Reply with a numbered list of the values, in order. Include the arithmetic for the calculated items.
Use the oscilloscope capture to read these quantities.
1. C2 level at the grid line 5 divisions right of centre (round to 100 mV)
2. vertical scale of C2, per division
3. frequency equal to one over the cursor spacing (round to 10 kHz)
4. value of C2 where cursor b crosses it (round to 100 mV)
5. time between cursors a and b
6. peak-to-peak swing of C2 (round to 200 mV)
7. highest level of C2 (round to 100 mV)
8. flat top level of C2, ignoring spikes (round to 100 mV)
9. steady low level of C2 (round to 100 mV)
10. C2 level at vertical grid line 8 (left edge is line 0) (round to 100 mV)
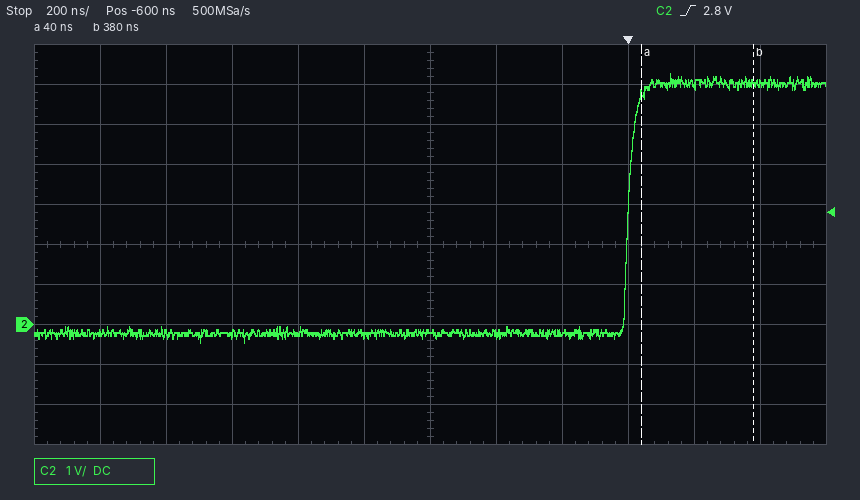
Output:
1. 6.0 V
2. 1 V
3. 1 / 340 ns ≈ 2.94 MHz
4. 6.0 V
5. 380 ns − (40 ns) = 340 ns
6. 6.8 V
7. 6.3 V
8. 6.0 V
9. -200 mV
10. -200 mV
